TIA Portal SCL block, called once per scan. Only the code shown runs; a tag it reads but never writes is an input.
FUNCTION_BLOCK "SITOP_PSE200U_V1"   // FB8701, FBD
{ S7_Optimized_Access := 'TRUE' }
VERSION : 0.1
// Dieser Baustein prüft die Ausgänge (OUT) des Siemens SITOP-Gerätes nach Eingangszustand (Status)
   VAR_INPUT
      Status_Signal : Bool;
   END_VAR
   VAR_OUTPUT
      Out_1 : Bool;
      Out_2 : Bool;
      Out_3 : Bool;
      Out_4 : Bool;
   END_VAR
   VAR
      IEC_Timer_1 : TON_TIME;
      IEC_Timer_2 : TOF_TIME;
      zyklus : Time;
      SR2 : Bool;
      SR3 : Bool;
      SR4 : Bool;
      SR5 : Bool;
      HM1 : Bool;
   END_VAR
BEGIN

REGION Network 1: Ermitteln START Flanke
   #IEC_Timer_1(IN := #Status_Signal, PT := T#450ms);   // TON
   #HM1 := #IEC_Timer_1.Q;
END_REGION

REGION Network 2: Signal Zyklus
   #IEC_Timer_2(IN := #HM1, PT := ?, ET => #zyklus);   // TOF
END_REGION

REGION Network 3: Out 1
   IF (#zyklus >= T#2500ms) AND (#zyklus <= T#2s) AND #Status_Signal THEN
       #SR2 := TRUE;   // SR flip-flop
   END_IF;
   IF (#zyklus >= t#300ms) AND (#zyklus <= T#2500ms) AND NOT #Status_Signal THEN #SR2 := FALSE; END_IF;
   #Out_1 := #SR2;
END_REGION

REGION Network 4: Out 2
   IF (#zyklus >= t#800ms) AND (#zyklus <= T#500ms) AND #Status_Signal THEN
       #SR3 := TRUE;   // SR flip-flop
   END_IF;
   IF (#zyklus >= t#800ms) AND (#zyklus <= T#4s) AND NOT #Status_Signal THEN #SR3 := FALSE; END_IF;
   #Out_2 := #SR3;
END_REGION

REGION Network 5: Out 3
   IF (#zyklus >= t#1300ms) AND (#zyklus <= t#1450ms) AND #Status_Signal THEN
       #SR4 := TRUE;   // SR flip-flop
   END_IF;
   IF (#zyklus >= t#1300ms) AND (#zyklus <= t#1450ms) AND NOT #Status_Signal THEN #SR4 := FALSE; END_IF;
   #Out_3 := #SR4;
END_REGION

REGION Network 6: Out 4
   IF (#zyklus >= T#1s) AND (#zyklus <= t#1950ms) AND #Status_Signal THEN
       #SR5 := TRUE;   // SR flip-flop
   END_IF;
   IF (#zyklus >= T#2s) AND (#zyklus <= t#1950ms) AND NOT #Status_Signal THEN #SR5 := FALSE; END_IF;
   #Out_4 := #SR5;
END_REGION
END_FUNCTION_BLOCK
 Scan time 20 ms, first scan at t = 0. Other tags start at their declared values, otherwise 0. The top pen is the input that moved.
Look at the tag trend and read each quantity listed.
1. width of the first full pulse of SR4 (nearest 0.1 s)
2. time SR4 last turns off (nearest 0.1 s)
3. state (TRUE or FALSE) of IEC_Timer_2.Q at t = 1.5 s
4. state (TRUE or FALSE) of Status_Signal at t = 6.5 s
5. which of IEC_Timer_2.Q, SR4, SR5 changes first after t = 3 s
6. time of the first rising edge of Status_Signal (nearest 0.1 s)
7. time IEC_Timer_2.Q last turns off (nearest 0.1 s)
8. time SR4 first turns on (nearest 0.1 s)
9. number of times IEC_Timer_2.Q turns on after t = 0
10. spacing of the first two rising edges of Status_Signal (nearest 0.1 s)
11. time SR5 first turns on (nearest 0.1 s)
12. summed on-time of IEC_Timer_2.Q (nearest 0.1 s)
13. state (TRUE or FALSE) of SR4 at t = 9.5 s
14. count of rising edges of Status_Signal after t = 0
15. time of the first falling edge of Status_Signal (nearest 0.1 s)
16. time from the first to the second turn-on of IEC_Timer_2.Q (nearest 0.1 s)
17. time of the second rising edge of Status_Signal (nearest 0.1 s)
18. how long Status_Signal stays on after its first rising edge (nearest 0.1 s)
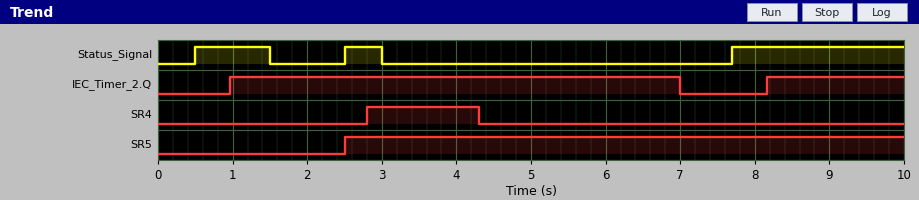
1.5 s
4.3 s
TRUE
FALSE
SR4
0.5 s
7.0 s
2.8 s
2
2.0 s
2.5 s
7.9 s
FALSE
3
1.5 s
7.2 s
2.5 s
1.0 s
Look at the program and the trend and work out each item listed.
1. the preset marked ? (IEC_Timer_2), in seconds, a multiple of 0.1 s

4.0 s
